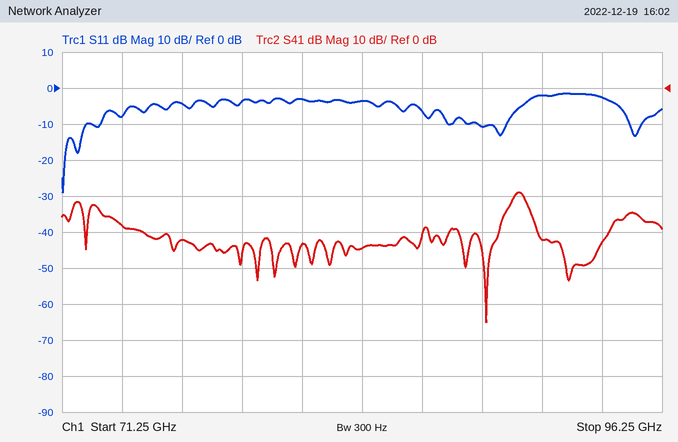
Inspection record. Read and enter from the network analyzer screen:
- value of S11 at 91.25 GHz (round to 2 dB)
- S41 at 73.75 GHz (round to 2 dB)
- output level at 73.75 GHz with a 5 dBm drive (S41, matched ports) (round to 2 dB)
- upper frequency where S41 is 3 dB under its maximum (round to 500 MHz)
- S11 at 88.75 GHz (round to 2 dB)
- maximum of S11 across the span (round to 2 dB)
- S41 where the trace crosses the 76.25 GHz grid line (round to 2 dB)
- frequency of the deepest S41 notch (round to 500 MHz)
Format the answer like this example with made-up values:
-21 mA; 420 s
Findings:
-2 dB; -38 dB; -34 dBm; 90.5 GHz; -10 dB; -2 dB; -42 dB; 89.0 GHz
